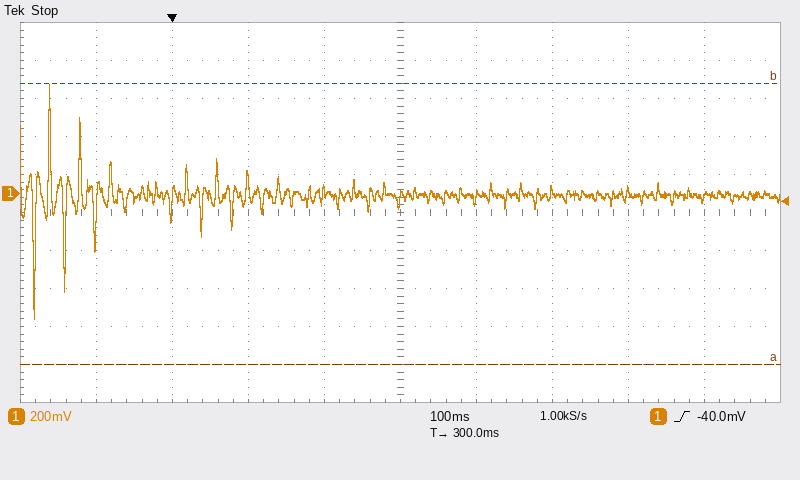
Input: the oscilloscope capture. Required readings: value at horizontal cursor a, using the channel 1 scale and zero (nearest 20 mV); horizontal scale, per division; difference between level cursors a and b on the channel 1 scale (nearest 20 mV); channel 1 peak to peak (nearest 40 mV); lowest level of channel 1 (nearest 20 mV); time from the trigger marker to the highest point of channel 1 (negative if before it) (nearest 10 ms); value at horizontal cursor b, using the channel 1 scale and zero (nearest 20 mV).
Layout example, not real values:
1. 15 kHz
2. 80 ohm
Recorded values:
1. -900 mV
2. 100 ms
3. 1.48 V
4. 1.24 V
5. -660 mV
6. -160 ms
7. 580 mV
